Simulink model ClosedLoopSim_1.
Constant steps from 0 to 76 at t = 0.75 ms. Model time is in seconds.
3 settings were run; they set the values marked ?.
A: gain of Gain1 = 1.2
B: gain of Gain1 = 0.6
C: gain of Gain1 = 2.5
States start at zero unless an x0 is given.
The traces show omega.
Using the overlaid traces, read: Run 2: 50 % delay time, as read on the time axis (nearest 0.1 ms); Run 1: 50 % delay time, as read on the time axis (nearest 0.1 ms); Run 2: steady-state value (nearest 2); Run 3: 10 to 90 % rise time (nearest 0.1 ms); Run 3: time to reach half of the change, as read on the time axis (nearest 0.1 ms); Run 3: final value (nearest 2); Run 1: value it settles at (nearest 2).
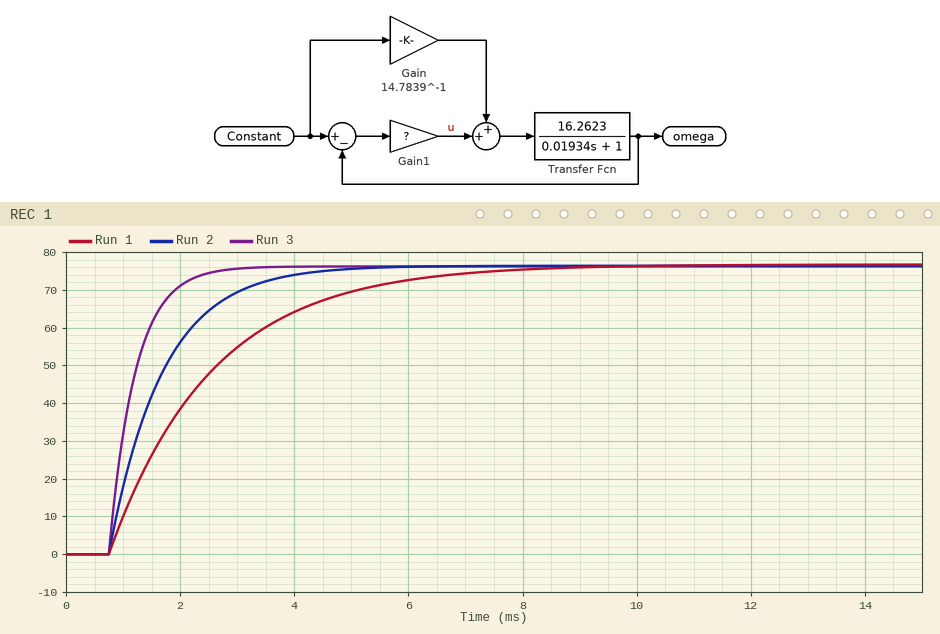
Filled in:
1.4 ms
2.0 ms
76
1.0 ms
1.1 ms
76
76
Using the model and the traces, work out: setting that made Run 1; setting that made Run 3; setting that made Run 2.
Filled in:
B
C
A
